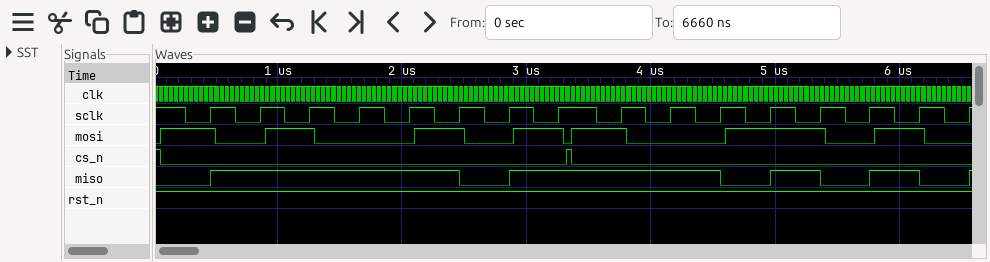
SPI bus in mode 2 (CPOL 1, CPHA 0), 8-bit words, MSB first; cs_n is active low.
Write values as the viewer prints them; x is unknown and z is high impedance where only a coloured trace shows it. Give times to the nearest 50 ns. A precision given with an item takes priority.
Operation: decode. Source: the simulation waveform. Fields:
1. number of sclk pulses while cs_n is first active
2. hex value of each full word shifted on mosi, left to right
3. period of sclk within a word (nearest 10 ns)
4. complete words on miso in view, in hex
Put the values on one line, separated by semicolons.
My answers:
8; A5, 9A; 400 ns; 7D, EA
